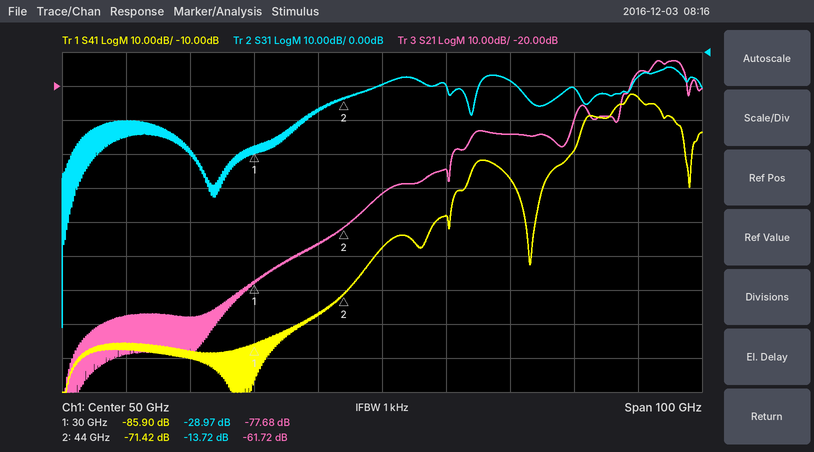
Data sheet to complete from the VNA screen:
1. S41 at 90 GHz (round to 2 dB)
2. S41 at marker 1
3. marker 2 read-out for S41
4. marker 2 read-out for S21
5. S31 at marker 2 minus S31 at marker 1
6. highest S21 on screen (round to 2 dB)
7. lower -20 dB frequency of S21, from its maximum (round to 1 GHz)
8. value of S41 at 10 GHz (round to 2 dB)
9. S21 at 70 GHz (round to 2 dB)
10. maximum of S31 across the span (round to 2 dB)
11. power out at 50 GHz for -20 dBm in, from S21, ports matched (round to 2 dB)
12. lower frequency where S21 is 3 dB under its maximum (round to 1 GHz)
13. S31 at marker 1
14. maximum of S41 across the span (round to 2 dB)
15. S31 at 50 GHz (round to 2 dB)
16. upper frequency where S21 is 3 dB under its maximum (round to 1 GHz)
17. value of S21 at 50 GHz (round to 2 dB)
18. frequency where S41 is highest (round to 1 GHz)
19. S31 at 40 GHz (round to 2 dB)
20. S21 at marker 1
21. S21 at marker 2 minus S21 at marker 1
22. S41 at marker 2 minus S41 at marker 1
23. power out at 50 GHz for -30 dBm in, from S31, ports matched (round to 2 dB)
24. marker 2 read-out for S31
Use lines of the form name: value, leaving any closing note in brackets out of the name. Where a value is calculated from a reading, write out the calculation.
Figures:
S41 at 90 GHz: -14 dB
S41 at marker 1: -85.90 dB
marker 2 read-out for S41: -71.42 dB
marker 2 read-out for S21: -61.72 dB
S31 at marker 2 minus S31 at marker 1: -13.72 − (-28.97) = 15.25 dB
highest S21 on screen: -12 dB
lower -20 dB frequency of S21, from its maximum: 80 GHz
value of S41 at 10 GHz: -86 dB
S21 at 70 GHz: -34 dB
maximum of S31 across the span: -4 dB
power out at 50 GHz for -20 dBm in, from S21, ports matched: -20 dBm + (-52 dB) = -72 dBm
lower frequency where S21 is 3 dB under its maximum: 92 GHz
S31 at marker 1: -28.97 dB
maximum of S41 across the span: -12 dB
S31 at 50 GHz: -10 dB
upper frequency where S21 is 3 dB under its maximum: 97 GHz
value of S21 at 50 GHz: -52 dB
frequency where S41 is highest: 89 GHz
S31 at 40 GHz: -18 dB
S21 at marker 1: -77.68 dB
S21 at marker 2 minus S21 at marker 1: -61.72 − (-77.68) = 15.96 dB
S41 at marker 2 minus S41 at marker 1: -71.42 − (-85.9) = 14.48 dB
power out at 50 GHz for -30 dBm in, from S31, ports matched: -30 dBm + (-10 dB) = -40 dBm
marker 2 read-out for S31: -13.72 dB
